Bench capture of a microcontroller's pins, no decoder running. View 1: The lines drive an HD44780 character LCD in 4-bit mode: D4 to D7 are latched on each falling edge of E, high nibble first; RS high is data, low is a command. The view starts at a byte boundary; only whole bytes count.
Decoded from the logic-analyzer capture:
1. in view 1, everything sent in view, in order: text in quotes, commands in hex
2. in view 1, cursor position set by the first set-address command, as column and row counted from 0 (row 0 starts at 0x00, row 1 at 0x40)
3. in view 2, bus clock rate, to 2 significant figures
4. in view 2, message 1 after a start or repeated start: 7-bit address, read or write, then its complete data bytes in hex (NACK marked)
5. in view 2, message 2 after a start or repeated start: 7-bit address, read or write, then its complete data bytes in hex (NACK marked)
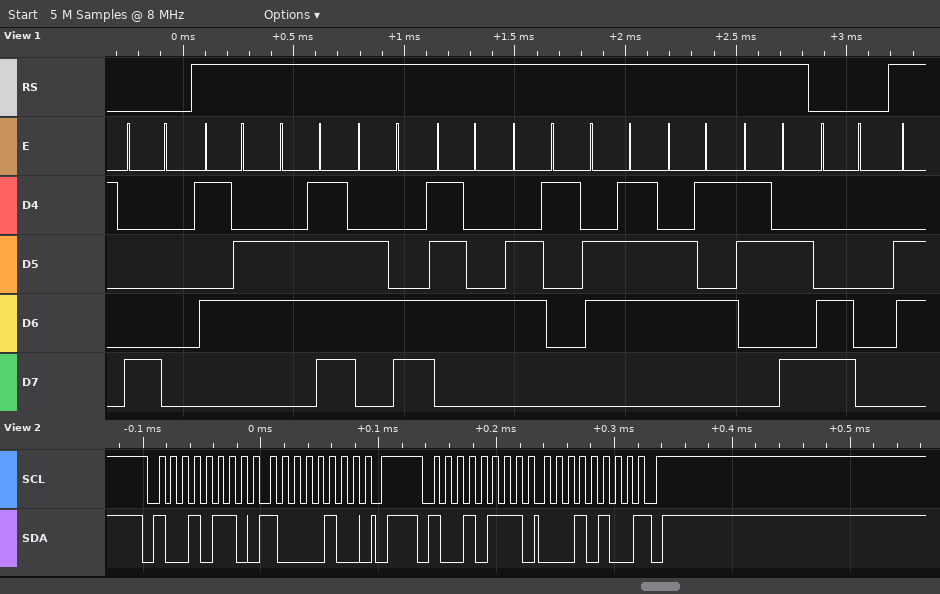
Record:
0x80 "Voltage:" 0xC0
column 0, row 0
100 kHz
0x4B write: 84
0x4B read: 14 NACK
